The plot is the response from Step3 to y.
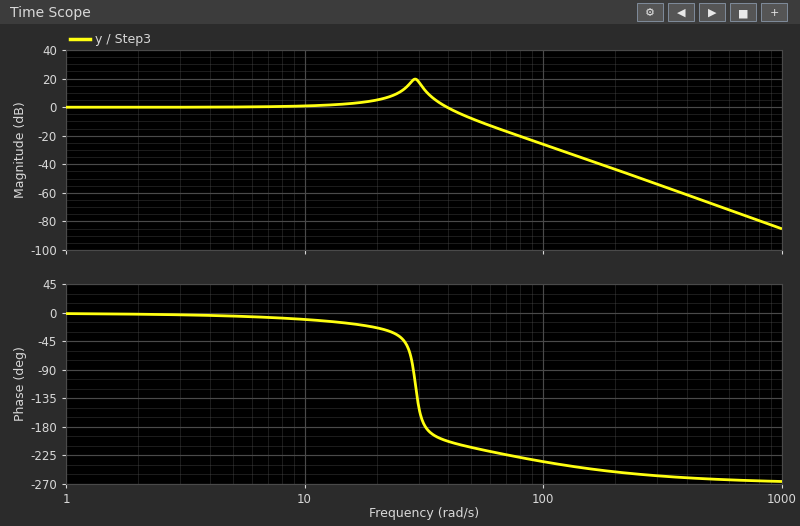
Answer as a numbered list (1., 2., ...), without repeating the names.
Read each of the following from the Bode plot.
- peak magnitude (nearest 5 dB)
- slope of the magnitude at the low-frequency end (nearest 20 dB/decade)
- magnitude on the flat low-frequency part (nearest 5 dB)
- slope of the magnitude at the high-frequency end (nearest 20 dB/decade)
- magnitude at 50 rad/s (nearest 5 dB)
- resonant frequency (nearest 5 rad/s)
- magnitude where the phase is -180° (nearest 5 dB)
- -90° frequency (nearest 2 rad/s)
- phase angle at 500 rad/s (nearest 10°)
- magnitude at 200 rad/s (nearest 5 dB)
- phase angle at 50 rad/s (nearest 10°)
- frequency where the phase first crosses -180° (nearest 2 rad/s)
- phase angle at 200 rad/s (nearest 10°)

1. 20 dB
2. 0 dB/decade
3. 0 dB
4. -60 dB/decade
5. -10 dB
6. 30 rad/s
7. 10 dB
8. 28 rad/s
9. -260°
10. -45 dB
11. -210°
12. 32 rad/s
13. -250°
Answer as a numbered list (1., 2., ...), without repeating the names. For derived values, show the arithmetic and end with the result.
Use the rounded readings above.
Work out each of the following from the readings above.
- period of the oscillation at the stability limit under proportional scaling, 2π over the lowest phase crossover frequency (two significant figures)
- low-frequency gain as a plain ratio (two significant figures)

1. 2π / 32 = 0.20 s
2. 10^(0 / 20) = 1.0
